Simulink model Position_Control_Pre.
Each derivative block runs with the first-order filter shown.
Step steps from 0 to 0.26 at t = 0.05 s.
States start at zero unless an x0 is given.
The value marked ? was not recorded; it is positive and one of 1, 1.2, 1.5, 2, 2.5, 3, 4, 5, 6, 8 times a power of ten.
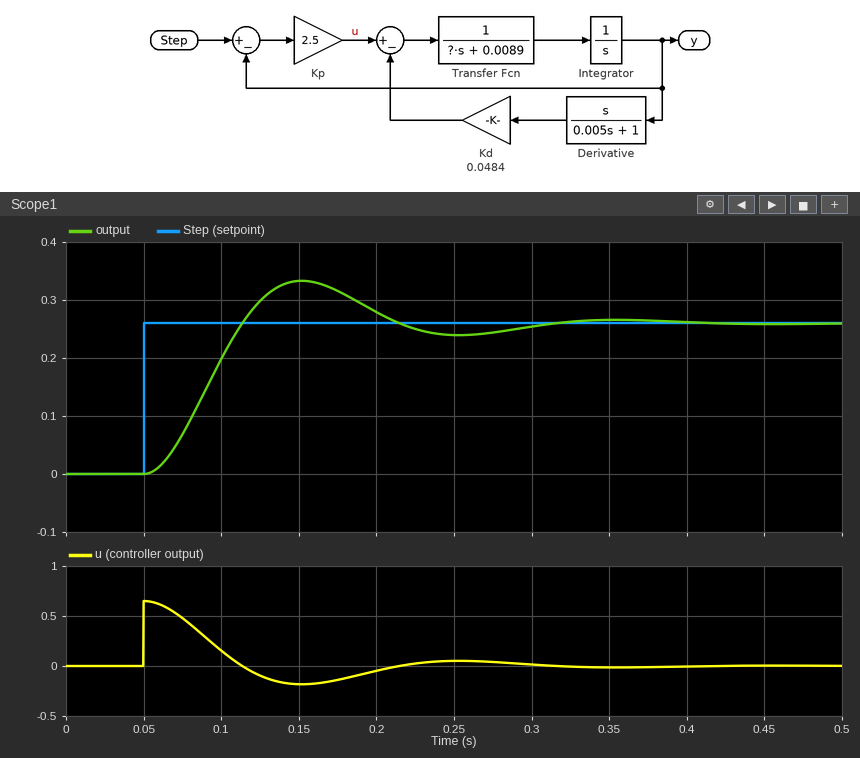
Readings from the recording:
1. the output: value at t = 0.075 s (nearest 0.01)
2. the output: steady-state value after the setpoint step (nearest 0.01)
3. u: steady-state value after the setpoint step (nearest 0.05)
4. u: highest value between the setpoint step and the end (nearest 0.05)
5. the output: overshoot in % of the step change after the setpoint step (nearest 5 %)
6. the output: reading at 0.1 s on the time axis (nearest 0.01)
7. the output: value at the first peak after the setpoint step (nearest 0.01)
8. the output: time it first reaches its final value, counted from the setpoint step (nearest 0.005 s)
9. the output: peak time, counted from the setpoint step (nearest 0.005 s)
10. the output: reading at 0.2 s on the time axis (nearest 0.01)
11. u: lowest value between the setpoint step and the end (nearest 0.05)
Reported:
0.07
0.26
0.00
0.65
30 %
0.20
0.33
0.065 s
0.100 s
0.28
-0.20
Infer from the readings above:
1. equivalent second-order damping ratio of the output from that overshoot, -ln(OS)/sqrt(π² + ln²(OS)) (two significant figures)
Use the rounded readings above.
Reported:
0.36
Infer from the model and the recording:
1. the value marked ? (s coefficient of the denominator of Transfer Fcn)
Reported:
0.0025
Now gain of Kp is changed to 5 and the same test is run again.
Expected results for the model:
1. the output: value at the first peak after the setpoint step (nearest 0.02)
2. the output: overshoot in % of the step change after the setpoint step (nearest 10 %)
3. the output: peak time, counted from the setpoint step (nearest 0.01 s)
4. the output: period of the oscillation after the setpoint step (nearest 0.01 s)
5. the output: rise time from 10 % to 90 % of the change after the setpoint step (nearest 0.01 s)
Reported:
0.38
40 %
0.07 s
0.14 s
0.03 s
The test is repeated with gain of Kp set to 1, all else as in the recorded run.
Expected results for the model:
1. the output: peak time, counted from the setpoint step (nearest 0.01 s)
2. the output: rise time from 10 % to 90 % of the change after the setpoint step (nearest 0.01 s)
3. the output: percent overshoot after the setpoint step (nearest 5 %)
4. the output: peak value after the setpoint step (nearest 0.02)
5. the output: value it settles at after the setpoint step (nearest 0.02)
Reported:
0.19 s
0.09 s
10 %
0.28
0.26
